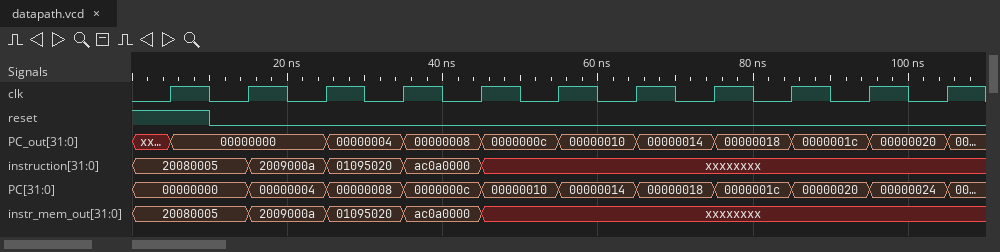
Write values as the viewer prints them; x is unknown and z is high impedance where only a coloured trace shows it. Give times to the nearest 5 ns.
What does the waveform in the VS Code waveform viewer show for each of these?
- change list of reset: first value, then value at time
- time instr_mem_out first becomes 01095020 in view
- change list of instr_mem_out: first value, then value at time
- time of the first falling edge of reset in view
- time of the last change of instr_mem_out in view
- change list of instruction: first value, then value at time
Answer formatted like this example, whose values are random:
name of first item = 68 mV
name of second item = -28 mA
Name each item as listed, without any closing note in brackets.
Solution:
change list of reset: first value, then value at time = 1, 0 at 10 ns
time instr_mem_out first becomes 01095020 in view = 25 ns
change list of instr_mem_out: first value, then value at time = 20080005, 2009000a at 15 ns, 01095020 at 25 ns, ac0a0000 at 35 ns, xxxxxxxx at 45 ns
time of the first falling edge of reset in view = 10 ns
time of the last change of instr_mem_out in view = 45 ns
change list of instruction: first value, then value at time = 20080005, 2009000a at 15 ns, 01095020 at 25 ns, ac0a0000 at 35 ns, xxxxxxxx at 45 ns
